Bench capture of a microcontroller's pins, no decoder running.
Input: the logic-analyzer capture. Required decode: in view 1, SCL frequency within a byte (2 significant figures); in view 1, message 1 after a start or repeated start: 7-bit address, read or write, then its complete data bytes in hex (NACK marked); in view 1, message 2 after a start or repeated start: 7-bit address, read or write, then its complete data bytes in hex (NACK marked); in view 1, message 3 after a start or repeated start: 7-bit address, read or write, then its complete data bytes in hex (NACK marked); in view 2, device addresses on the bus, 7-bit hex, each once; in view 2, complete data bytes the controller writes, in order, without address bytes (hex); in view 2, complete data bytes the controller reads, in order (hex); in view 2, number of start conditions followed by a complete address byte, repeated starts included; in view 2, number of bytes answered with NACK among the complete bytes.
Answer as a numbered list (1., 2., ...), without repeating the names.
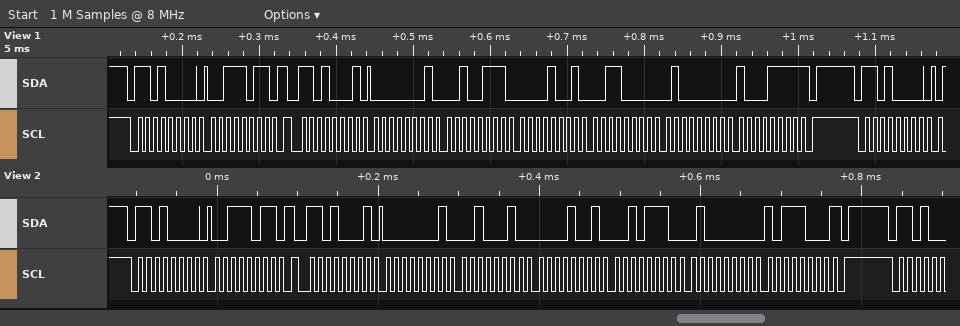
1. 100 kHz
2. 0x68 write: 3B
3. 0x68 read: 01 27 09 30 40 8F NACK
4. 0x68 write
5. 0x68
6. 3B
7. 01 22 09 2E 40 B8
8. 2
9. 1
